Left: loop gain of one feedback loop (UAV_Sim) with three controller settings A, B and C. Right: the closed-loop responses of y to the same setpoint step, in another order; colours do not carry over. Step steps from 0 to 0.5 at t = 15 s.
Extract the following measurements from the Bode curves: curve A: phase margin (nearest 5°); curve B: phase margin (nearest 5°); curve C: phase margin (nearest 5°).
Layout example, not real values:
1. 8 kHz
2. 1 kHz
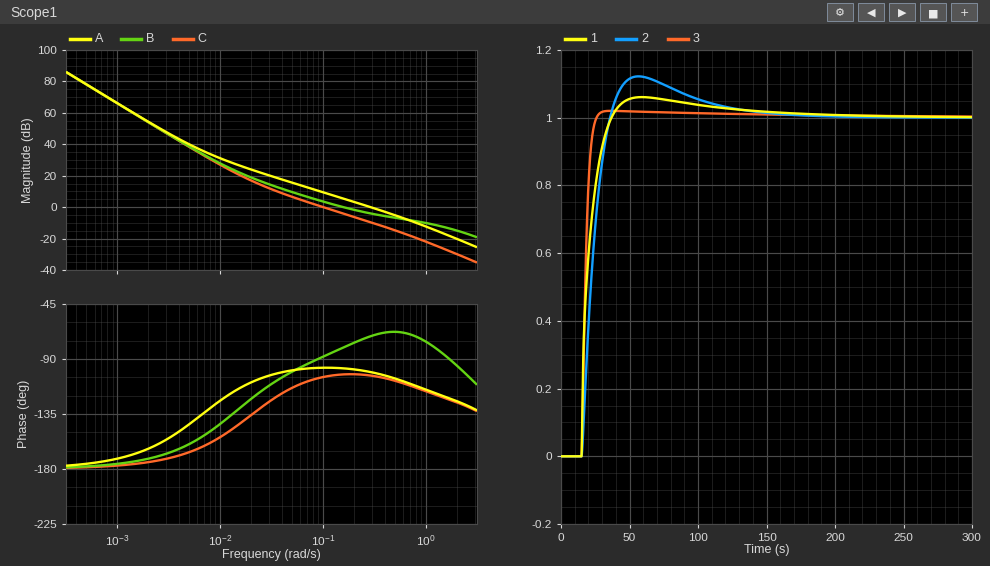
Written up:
1. 80°
2. 100°
3. 75°
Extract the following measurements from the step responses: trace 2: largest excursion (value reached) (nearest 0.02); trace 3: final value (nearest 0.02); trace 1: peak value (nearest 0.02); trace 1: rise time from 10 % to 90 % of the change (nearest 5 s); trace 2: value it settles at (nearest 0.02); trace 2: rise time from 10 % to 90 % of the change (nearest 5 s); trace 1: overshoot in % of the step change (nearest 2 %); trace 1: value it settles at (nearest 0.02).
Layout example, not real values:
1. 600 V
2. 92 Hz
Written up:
1. 1.12
2. 1.00
3. 1.06
4. 15 s
5. 1.00
6. 15 s
7. 6 %
8. 1.00
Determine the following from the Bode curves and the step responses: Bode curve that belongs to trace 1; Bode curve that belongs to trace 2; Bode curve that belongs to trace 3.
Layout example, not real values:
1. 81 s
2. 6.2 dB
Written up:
1. B
2. C
3. A
